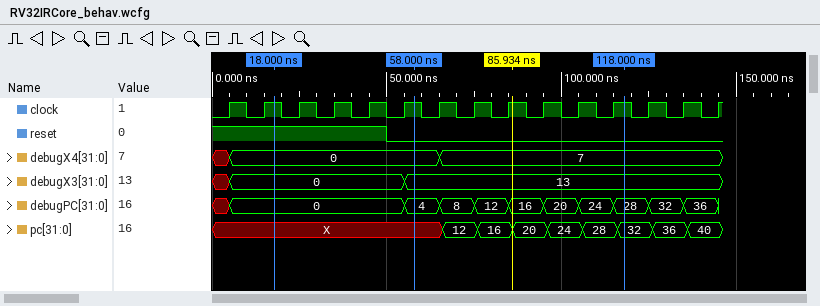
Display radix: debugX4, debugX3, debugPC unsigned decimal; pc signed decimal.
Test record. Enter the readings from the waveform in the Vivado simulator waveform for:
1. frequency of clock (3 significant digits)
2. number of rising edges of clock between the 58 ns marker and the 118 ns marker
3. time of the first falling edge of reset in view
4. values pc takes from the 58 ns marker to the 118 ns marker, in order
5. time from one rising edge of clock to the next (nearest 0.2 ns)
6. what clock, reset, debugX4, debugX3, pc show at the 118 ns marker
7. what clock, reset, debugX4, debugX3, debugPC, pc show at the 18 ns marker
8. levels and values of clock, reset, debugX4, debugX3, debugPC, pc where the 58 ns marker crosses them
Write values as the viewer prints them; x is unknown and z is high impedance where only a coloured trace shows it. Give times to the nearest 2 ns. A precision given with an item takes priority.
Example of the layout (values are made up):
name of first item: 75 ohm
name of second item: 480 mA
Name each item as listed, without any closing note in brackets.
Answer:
frequency of clock: 100 MHz
number of rising edges of clock between the 58 ns marker and the 118 ns marker: 6
time of the first falling edge of reset in view: 50 ns
values pc takes from the 58 ns marker to the 118 ns marker, in order: X, 12, 16, 20, 24, 28, 32
time from one rising edge of clock to the next: 10 ns
what clock, reset, debugX4, debugX3, pc show at the 118 ns marker: clock=1, reset=0, debugX4=7, debugX3=13, pc=32
what clock, reset, debugX4, debugX3, debugPC, pc show at the 18 ns marker: clock=1, reset=1, debugX4=0, debugX3=0, debugPC=0, pc=X
levels and values of clock, reset, debugX4, debugX3, debugPC, pc where the 58 ns marker crosses them: clock=1, reset=0, debugX4=0, debugX3=13, debugPC=4, pc=X
